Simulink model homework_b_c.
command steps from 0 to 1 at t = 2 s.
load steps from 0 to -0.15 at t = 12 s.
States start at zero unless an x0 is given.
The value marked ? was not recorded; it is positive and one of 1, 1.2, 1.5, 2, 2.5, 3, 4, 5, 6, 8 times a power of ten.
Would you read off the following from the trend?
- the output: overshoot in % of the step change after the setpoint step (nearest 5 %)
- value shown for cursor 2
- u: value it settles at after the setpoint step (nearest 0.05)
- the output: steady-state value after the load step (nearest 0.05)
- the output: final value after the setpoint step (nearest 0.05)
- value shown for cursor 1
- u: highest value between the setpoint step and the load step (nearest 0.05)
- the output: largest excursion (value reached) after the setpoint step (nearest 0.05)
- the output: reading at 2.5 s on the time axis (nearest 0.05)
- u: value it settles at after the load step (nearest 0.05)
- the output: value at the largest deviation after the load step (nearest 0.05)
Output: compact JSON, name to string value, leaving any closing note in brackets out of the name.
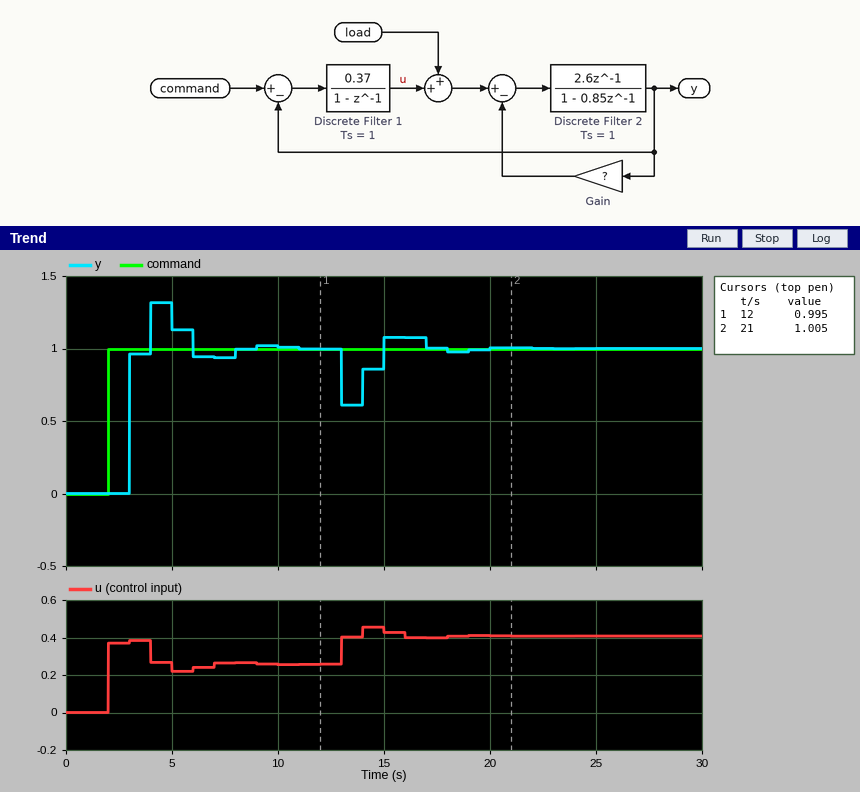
{"the output: overshoot in % of the step change after the setpoint step": "30 %", "value shown for cursor 2": "1.005", "u: value it settles at after the setpoint step": "0.25", "the output: steady-state value after the load step": "1.00", "the output: final value after the setpoint step": "1.00", "value shown for cursor 1": "0.995", "u: highest value between the setpoint step and the load step": "0.40", "the output: largest excursion (value reached) after the setpoint step": "1.30", "the output: reading at 2.5 s on the time axis": "0.00", "u: value it settles at after the load step": "0.40", "the output: value at the largest deviation after the load step": "0.60"}
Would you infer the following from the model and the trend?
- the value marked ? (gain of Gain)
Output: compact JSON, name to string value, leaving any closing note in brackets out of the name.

{"the value marked ?": "0.2"}
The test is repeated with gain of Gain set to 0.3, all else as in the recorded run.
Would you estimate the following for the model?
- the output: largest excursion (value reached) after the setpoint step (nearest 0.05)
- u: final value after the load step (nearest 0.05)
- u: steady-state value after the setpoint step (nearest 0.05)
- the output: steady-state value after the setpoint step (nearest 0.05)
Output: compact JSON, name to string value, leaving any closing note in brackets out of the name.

{"the output: largest excursion (value reached) after the setpoint step": "1.05", "u: final value after the load step": "0.50", "u: steady-state value after the setpoint step": "0.35", "the output: steady-state value after the setpoint step": "1.00"}
